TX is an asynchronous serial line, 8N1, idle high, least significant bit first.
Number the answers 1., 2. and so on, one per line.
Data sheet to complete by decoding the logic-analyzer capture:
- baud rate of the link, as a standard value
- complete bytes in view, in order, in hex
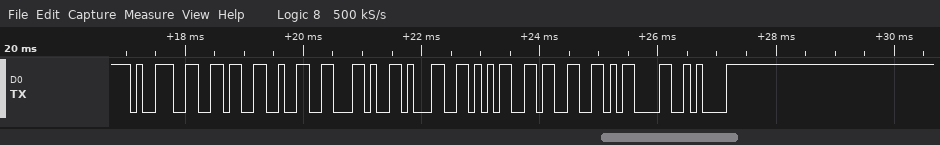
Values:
1. 9600 baud
2. 0x39 0x36 0x32 0x2C 0x31 0x35 0x33 0x0D 0x0A
